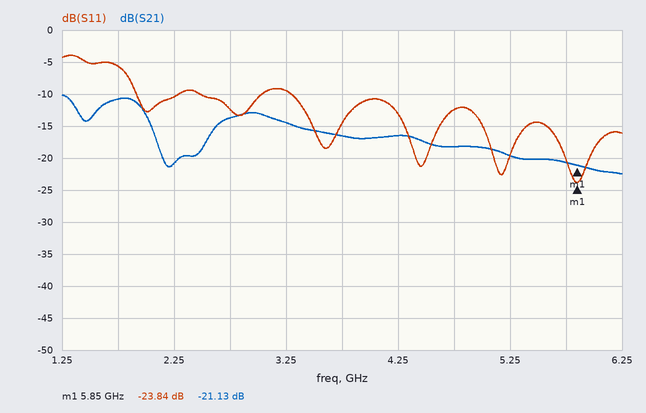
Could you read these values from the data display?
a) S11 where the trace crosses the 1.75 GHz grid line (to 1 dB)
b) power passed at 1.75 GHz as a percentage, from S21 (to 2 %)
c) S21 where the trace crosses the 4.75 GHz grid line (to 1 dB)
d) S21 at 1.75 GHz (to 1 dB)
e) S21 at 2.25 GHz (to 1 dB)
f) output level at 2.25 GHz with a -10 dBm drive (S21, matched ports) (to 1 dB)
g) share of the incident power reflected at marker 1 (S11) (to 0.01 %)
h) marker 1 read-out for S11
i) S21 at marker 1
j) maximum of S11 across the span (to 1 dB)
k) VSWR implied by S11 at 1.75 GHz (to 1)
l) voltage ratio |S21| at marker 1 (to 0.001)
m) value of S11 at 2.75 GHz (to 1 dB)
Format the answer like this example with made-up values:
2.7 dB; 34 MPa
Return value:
-6 dB; 8 %; -18 dB; -11 dB; -21 dB; -31 dBm; 0.41 %; -23.84 dB; -21.13 dB; -4 dB; 3; 0.088; -12 dB
